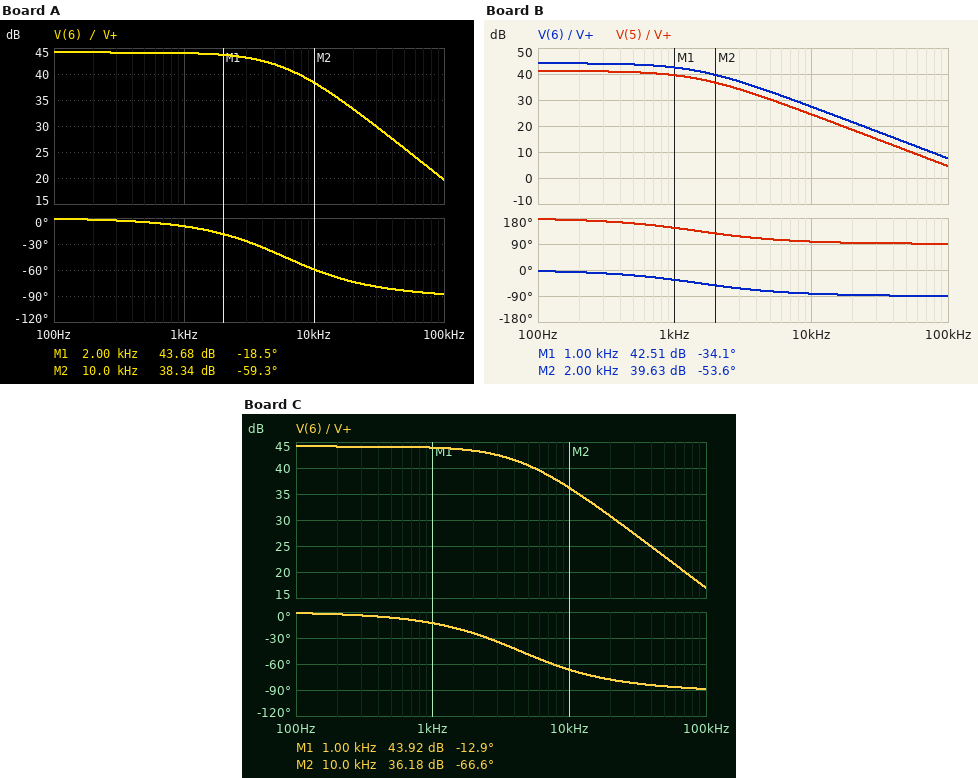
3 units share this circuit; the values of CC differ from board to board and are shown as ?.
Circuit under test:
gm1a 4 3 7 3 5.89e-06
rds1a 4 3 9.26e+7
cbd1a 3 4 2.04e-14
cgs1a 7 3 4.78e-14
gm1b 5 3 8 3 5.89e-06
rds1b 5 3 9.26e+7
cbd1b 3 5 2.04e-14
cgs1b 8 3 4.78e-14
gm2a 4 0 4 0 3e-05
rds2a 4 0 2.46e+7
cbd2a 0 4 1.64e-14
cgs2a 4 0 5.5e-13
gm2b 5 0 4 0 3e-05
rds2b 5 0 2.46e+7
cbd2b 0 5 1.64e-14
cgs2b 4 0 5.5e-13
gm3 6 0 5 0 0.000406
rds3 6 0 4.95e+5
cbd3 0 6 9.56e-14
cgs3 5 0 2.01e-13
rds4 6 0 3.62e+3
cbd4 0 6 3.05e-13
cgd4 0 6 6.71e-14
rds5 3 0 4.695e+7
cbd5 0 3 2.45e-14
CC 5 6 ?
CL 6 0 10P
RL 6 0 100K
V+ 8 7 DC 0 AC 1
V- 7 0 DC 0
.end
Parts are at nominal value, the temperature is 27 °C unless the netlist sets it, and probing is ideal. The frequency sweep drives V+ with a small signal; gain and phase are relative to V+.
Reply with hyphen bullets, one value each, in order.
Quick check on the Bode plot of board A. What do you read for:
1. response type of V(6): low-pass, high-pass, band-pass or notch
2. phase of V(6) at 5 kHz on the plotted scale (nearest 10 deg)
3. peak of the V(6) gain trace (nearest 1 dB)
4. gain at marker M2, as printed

- low-pass
- -40 deg
- 44 dB
- 38.34 dB
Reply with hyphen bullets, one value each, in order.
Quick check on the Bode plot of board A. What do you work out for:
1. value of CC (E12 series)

- 470 fF
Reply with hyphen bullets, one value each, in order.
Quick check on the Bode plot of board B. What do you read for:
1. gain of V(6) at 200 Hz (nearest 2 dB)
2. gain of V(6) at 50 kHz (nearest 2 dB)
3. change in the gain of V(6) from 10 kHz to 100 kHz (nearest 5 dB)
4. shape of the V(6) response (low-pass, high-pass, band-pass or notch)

- 44 dB
- 14 dB
- -20 dB
- low-pass
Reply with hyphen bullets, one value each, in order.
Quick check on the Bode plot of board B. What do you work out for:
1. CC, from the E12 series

- 2.2 pF
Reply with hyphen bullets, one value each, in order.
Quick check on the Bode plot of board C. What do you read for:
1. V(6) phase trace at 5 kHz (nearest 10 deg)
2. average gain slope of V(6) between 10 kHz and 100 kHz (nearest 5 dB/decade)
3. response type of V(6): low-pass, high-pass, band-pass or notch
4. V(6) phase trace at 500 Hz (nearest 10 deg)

- -50 deg
- -20 dB/decade
- low-pass
- -10 deg
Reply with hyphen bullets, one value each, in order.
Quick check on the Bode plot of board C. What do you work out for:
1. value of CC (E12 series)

- 680 fF
